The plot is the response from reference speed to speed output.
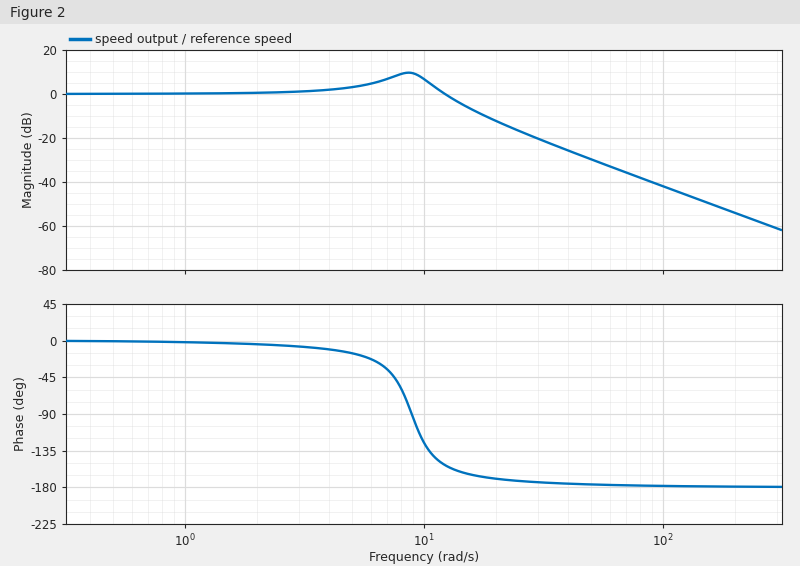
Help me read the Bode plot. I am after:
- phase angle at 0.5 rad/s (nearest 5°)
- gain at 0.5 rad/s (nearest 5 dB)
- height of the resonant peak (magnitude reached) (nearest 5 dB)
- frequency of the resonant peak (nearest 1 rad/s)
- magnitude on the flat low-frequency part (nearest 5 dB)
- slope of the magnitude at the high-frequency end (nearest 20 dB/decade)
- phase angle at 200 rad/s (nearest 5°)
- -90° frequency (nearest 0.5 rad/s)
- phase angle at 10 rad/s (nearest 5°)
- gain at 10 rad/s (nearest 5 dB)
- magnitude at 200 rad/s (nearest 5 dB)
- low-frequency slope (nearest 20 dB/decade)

0°
0 dB
10 dB
9 rad/s
0 dB
-40 dB/decade
-180°
9.0 rad/s
-125°
5 dB
-55 dB
0 dB/decade
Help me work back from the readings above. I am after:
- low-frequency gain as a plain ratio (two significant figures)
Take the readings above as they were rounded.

1.0
